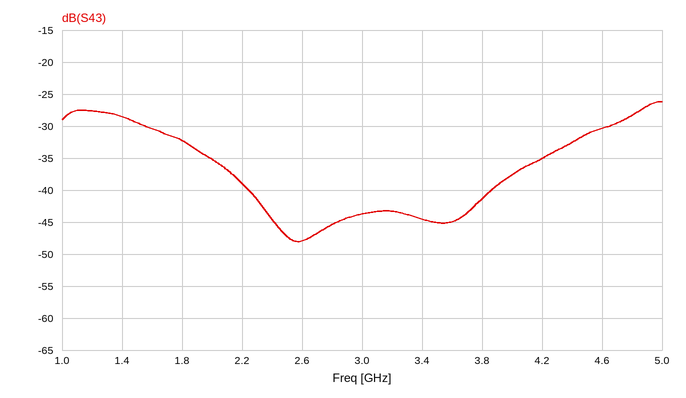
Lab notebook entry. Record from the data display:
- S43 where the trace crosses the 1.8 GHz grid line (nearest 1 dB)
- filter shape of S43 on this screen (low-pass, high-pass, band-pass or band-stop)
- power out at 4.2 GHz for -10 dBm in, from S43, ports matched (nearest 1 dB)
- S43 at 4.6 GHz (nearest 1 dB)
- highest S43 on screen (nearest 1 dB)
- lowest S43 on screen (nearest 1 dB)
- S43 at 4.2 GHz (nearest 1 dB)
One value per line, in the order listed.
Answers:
-32 dB
band-stop
-45 dBm
-30 dB
-26 dB
-48 dB
-35 dB
